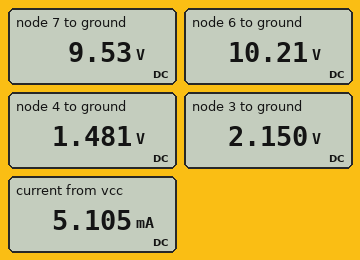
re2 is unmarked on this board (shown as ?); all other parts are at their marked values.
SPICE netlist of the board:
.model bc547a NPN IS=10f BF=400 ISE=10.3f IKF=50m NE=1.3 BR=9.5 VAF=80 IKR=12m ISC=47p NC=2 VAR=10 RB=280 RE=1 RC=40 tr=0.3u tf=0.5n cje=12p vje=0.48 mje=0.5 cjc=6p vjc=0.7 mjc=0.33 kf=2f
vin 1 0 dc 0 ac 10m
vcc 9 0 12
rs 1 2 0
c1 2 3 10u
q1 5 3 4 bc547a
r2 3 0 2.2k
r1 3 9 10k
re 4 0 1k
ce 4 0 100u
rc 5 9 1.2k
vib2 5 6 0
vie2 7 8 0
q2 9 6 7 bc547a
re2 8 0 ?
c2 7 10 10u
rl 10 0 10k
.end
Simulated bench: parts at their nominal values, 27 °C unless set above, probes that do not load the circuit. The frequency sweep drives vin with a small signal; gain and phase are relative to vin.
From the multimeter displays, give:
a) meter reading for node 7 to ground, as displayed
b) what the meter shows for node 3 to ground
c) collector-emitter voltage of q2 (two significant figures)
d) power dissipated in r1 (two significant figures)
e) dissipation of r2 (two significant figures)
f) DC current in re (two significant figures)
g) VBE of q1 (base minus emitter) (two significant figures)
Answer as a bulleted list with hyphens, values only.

- 9.53 V
- 2.150 V
- 2.5 V
- 9.7 mW
- 2.1 mW
- 1.5 mA
- 670 mV
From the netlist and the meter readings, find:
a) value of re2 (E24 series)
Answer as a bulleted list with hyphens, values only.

- 3.6 kΩ
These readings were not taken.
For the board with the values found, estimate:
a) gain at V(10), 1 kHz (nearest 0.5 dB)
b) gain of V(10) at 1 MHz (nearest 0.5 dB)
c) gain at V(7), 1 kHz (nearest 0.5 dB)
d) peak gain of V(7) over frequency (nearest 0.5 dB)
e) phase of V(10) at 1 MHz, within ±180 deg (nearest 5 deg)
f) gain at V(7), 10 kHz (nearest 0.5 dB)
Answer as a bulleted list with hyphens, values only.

- 35.0 dB
- 34.5 dB
- 35.0 dB
- 35.0 dB
- 155 deg
- 35.0 dB
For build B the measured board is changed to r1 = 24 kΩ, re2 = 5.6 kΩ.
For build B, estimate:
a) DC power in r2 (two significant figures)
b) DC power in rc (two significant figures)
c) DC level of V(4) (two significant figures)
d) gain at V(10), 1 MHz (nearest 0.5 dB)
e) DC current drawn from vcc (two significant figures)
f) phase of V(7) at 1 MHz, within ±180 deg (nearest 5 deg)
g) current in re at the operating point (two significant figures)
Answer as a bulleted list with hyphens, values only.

- 460 µW
- 180 µW
- 370 mV
- 24.0 dB
- 2.8 mA
- 170 deg
- 370 µA
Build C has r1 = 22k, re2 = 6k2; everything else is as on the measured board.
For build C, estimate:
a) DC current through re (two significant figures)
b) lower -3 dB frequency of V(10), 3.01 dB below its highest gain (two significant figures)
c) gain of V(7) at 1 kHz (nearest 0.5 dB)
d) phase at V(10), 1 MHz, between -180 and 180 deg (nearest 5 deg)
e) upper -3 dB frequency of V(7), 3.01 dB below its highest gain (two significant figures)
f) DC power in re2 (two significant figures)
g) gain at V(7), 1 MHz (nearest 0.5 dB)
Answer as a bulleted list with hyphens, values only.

- 450 µA
- 31 Hz
- 26.0 dB
- 165 deg
- 5.0 MHz
- 19 mW
- 25.5 dB
